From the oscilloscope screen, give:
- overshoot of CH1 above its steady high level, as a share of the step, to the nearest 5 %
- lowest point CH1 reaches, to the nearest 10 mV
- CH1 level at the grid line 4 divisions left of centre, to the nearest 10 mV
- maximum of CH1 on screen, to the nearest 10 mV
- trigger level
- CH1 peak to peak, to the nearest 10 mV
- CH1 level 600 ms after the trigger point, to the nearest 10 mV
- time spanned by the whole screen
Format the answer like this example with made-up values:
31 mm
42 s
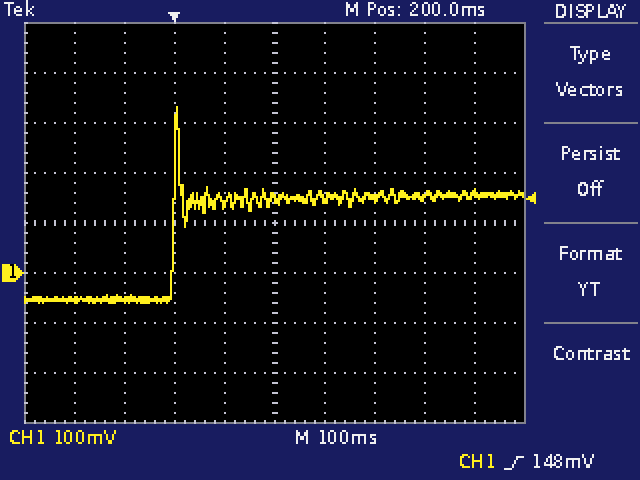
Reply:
85 %
-60 mV
-50 mV
330 mV
148 mV
390 mV
160 mV
1 s
